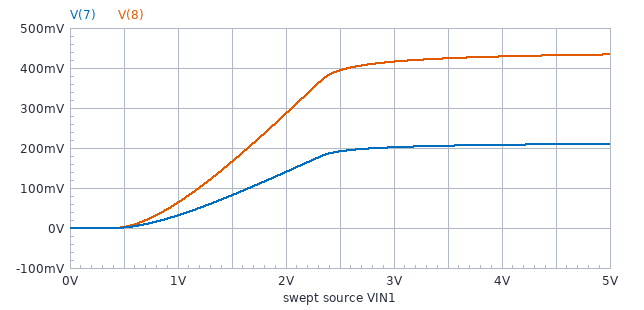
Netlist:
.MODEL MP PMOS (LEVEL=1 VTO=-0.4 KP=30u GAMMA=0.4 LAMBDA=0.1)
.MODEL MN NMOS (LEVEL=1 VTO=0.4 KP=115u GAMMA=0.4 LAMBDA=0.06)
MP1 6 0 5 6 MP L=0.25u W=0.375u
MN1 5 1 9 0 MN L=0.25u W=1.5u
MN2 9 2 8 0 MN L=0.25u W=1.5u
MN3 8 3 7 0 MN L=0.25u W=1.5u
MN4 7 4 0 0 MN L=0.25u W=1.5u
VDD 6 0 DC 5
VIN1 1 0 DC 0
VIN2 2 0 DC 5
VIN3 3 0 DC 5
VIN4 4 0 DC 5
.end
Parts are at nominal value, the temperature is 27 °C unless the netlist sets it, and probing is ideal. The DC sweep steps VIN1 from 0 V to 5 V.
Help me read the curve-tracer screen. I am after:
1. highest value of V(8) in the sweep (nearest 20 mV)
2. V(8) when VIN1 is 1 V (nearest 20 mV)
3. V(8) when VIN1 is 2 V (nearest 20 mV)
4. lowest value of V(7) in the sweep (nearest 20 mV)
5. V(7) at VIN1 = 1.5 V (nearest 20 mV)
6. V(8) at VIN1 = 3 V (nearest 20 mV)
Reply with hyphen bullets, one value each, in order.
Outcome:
- 440 mV
- 60 mV
- 280 mV
- 0 V
- 80 mV
- 420 mV
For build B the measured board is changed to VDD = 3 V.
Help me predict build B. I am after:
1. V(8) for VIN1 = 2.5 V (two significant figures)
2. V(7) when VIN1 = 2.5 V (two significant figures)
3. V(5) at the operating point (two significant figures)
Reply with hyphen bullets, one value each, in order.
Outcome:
- 120 mV
- 61 mV
- 3.0 V
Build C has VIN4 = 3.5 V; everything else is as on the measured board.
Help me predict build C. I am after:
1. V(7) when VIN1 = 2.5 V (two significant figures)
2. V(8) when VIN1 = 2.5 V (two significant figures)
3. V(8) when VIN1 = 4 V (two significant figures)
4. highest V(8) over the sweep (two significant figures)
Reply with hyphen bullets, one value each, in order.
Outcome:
- 280 mV
- 480 mV
- 530 mV
- 540 mV
